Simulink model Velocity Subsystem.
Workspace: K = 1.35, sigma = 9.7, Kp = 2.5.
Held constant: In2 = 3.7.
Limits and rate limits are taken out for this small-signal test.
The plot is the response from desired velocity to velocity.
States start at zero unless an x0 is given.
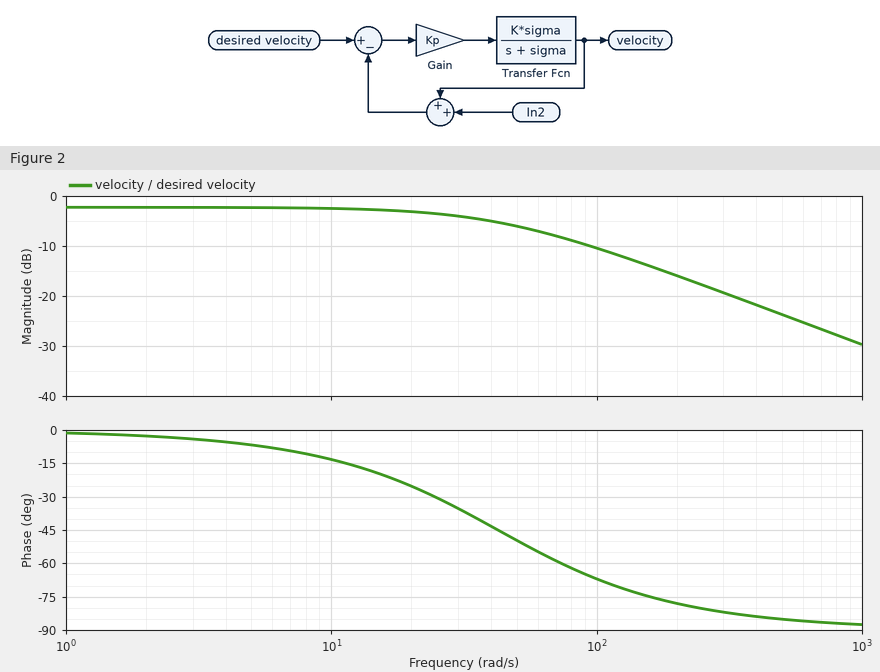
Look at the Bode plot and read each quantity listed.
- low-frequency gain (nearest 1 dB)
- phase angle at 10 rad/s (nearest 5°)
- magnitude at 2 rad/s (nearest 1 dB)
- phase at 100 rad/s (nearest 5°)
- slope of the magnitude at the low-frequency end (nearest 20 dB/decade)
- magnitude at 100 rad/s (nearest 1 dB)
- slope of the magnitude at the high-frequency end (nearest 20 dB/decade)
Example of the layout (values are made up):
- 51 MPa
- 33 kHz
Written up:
- -2 dB
- -15°
- -2 dB
- -65°
- 0 dB/decade
- -10 dB
- -20 dB/decade
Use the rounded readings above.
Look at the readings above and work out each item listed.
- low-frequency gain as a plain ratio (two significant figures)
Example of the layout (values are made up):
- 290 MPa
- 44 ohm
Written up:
- 0.79
